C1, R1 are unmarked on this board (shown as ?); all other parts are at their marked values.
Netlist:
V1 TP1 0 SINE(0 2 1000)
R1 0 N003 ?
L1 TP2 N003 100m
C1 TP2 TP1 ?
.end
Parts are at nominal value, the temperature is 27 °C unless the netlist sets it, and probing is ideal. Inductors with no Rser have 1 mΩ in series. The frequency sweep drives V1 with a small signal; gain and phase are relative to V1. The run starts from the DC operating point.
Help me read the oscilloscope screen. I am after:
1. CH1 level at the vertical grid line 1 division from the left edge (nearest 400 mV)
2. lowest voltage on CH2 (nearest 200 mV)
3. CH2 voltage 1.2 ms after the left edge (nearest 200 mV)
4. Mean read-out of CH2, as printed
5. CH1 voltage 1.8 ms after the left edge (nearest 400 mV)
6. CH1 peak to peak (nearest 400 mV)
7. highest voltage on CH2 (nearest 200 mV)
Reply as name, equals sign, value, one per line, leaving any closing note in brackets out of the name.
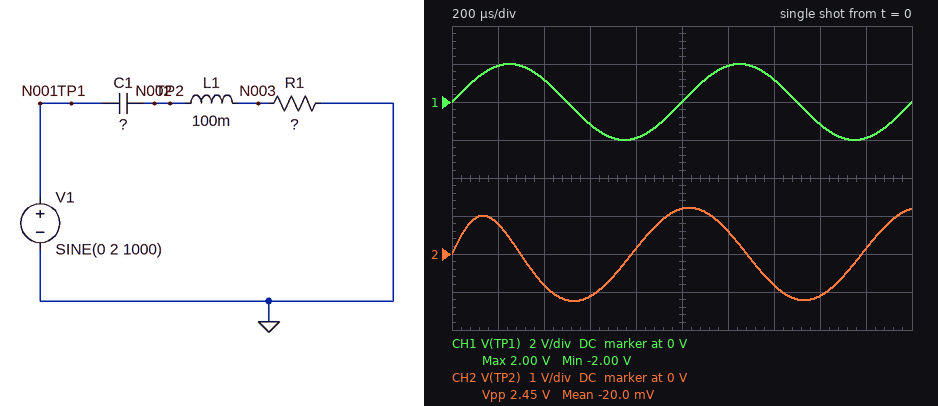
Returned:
CH1 level at the vertical grid line 1 division from the left edge = 2.0 V
lowest voltage on CH2 = -1.2 V
CH2 voltage 1.2 ms after the left edge = 600 mV
Mean read-out of CH2, as printed = -20.0 mV
CH1 voltage 1.8 ms after the left edge = -2.0 V
CH1 peak to peak = 4.0 V
highest voltage on CH2 = 1.2 V
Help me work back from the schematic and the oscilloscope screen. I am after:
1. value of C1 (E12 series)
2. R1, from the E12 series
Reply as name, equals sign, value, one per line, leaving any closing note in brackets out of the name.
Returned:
value of C1 = 56 nF
R1, from the E12 series = 1.5 kΩ
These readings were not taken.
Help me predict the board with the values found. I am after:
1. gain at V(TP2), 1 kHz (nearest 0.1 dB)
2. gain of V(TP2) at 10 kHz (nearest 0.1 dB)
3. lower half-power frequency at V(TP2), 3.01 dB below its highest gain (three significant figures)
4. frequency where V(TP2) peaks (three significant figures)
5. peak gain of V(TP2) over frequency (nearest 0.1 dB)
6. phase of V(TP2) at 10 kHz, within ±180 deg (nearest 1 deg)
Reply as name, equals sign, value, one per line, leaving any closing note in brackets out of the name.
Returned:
gain at V(TP2), 1 kHz = -4.3 dB
gain of V(TP2) at 10 kHz = 0.4 dB
lower half-power frequency at V(TP2), 3.01 dB below its highest gain = 1.48 kHz
frequency where V(TP2) peaks = 2.55 kHz
peak gain of V(TP2) over frequency = 2.9 dB
phase of V(TP2) at 10 kHz, within ±180 deg = 1 deg
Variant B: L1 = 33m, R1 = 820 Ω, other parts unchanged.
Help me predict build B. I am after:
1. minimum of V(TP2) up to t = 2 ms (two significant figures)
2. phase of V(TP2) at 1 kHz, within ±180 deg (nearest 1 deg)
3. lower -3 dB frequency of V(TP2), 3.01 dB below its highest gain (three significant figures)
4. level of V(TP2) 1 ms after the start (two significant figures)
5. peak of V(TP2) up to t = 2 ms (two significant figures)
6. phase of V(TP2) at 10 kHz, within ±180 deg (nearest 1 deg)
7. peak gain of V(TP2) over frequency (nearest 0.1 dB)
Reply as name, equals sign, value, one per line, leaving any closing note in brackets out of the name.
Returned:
minimum of V(TP2) up to t = 2 ms = -610 mV
phase of V(TP2) at 1 kHz, within ±180 deg = 87 deg
lower -3 dB frequency of V(TP2), 3.01 dB below its highest gain = 2.63 kHz
level of V(TP2) 1 ms after the start = 610 mV
peak of V(TP2) up to t = 2 ms = 650 mV
phase of V(TP2) at 10 kHz, within ±180 deg = 3 deg
peak gain of V(TP2) over frequency = 3.1 dB
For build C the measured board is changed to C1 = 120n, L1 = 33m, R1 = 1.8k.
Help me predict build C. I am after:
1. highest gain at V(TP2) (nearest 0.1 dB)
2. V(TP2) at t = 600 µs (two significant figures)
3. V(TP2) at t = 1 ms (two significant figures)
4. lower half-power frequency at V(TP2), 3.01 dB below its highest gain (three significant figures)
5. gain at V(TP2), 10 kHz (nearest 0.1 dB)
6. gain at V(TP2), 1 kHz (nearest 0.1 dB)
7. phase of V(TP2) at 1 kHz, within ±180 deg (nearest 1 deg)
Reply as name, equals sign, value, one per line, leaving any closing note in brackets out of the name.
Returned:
highest gain at V(TP2) = 0.5 dB
V(TP2) at t = 600 µs = -1.7 V
V(TP2) at t = 1 ms = 1.1 V
lower half-power frequency at V(TP2), 3.01 dB below its highest gain = 756 Hz
gain at V(TP2), 10 kHz = 0.3 dB
gain at V(TP2), 1 kHz = -1.4 dB
phase of V(TP2) at 1 kHz, within ±180 deg = 38 deg
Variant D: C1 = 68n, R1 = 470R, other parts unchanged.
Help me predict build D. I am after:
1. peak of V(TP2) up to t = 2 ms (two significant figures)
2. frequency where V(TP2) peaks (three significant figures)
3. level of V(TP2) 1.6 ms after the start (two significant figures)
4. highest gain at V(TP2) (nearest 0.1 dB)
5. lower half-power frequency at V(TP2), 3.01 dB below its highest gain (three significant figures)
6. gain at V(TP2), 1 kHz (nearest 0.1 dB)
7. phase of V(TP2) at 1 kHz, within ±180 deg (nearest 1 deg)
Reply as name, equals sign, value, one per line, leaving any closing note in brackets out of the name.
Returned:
peak of V(TP2) up to t = 2 ms = 960 mV
frequency where V(TP2) peaks = 2.00 kHz
level of V(TP2) 1.6 ms after the start = -260 mV
highest gain at V(TP2) = 9.0 dB
lower half-power frequency at V(TP2), 3.01 dB below its highest gain = 1.68 kHz
gain at V(TP2), 1 kHz = -7.1 dB
phase of V(TP2) at 1 kHz, within ±180 deg = 128 deg
